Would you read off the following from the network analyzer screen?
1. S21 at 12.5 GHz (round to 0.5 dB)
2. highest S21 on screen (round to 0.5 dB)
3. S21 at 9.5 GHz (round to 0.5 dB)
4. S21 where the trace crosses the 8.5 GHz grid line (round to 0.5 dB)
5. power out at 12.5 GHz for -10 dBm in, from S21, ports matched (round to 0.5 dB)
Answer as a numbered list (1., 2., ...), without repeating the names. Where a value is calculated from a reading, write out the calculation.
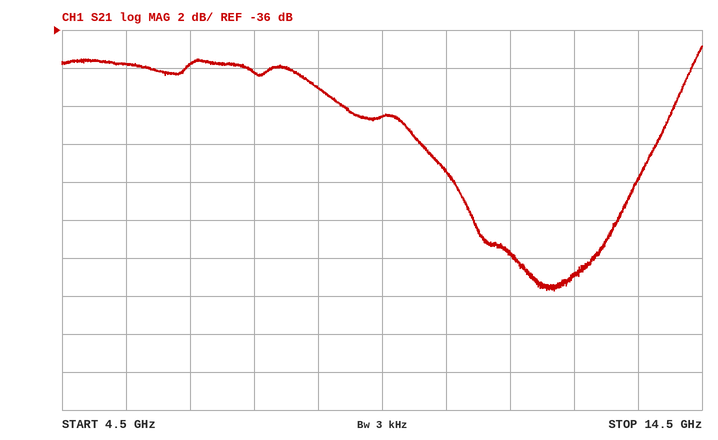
1. -49.0 dB
2. -37.0 dB
3. -40.5 dB
4. -39.0 dB
5. -10 dBm + (-49.0 dB) = -59.0 dBm
